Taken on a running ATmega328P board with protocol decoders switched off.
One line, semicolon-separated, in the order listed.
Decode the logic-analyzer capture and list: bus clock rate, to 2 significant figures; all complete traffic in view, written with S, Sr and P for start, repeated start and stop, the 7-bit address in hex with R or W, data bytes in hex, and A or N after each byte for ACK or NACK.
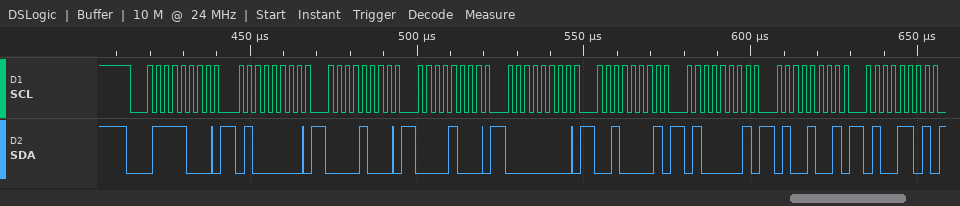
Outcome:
400 kHz; S 3CW A 40 A 08 A 08 A 00 A 21 A 41 A 49 A 4D A
